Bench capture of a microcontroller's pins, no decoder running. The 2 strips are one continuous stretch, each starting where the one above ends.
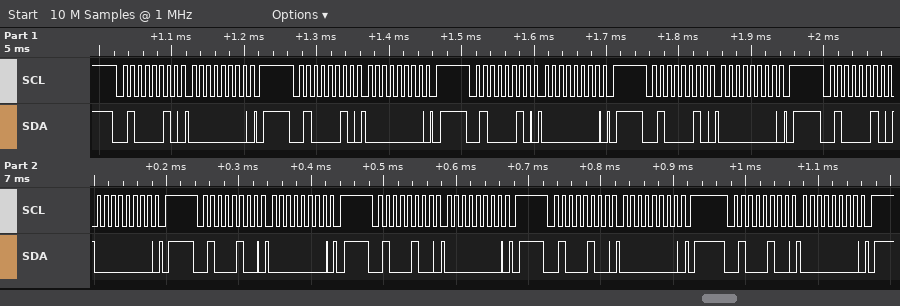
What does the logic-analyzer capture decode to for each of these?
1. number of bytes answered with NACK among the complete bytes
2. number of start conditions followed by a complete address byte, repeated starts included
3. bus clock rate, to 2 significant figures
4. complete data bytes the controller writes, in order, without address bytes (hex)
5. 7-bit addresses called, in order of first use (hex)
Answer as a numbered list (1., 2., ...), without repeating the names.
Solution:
1. 0
2. 9
3. 100 kHz
4. 00 00 00 00 00 00 00 00 00
5. 0x21 0x22
